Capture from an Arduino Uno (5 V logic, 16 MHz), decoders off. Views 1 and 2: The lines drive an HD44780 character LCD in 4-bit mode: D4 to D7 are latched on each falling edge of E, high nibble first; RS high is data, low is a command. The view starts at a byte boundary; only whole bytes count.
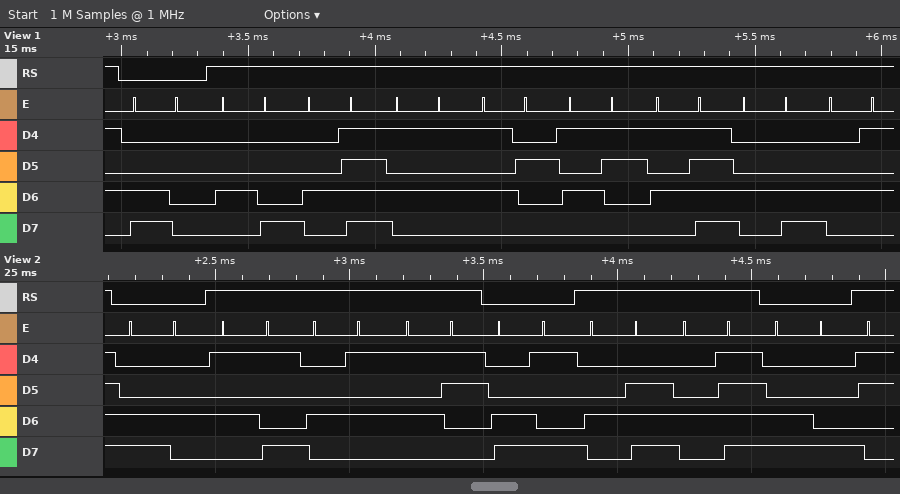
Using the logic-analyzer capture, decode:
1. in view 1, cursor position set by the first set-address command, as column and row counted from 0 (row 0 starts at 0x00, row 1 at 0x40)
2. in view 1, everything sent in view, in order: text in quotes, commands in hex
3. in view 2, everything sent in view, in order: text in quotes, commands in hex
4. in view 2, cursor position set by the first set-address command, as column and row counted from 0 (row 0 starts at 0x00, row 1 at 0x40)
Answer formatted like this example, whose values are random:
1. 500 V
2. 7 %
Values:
1. column 0, row 1
2. 0xC0 "HOURS_LE"
3. 0xC4 "YES" 0xC9 "NO" 0xC8
4. column 4, row 1
